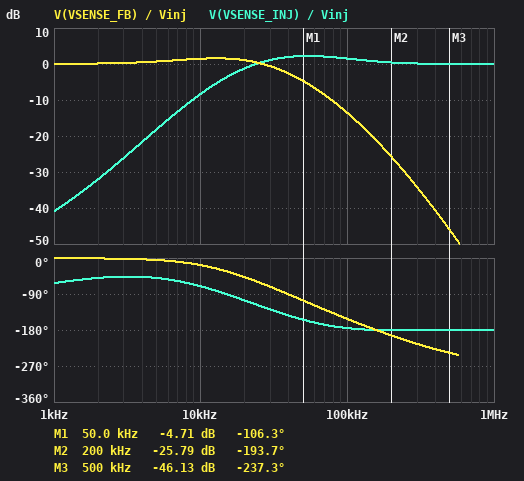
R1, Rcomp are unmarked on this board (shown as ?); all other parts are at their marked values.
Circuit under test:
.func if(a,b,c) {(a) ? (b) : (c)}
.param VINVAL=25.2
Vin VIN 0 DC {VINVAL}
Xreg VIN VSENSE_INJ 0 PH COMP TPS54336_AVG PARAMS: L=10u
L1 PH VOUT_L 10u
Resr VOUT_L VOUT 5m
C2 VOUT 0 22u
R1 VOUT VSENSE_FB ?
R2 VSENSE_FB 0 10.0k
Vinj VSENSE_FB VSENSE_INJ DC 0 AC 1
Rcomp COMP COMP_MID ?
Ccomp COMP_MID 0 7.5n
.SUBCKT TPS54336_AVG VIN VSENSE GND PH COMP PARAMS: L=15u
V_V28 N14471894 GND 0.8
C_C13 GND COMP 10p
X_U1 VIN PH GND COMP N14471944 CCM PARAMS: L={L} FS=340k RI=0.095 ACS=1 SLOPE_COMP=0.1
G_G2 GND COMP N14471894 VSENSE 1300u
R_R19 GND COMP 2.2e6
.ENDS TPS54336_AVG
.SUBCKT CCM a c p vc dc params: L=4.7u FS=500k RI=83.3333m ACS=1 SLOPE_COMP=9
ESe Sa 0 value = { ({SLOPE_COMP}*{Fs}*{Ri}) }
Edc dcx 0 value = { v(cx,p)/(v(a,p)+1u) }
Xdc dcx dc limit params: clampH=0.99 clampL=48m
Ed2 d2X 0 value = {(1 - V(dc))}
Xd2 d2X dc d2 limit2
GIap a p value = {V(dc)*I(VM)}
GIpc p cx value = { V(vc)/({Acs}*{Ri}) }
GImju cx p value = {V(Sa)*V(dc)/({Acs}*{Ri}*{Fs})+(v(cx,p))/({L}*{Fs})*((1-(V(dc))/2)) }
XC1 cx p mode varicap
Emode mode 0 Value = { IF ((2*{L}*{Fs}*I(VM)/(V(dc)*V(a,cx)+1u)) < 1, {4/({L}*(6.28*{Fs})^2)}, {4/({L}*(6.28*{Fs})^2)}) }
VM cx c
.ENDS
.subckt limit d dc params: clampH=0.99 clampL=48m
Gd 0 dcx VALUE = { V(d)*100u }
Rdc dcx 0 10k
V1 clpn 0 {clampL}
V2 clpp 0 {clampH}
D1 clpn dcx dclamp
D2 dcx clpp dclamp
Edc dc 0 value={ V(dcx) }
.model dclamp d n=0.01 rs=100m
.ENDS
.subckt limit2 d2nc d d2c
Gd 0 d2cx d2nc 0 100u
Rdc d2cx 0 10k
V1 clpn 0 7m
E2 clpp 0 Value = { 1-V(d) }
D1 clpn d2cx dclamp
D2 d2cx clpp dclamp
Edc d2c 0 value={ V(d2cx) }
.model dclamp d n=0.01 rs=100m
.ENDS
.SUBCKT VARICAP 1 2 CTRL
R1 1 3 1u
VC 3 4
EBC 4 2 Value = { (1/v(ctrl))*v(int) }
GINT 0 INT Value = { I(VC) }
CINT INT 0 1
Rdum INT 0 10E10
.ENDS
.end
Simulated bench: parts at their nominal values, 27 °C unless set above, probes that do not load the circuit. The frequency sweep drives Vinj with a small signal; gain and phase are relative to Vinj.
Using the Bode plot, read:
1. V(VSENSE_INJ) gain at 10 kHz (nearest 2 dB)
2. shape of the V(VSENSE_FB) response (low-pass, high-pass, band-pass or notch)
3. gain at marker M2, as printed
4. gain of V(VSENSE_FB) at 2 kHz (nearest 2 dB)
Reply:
-8 dB
low-pass
-25.79 dB
0 dB
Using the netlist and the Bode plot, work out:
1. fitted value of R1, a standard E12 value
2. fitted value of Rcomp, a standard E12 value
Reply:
100 kΩ
2.7 kΩ
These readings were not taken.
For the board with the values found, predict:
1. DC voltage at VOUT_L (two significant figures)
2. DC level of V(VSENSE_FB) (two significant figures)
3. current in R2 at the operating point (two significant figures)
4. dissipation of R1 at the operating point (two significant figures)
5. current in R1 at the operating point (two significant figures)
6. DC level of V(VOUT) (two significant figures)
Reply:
8.8 V
800 mV
80 µA
640 µW
80 µA
8.8 V
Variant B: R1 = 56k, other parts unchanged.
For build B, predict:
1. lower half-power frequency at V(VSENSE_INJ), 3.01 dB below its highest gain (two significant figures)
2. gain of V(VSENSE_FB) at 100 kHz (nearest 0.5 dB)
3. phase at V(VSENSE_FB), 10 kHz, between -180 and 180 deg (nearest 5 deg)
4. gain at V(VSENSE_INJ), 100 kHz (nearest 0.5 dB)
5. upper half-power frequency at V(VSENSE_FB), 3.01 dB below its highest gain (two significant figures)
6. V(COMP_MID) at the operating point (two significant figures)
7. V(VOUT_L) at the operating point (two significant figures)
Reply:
34 kHz
-9.5 dB
-10 deg
2.5 dB
59 kHz
130 mV
5.3 V
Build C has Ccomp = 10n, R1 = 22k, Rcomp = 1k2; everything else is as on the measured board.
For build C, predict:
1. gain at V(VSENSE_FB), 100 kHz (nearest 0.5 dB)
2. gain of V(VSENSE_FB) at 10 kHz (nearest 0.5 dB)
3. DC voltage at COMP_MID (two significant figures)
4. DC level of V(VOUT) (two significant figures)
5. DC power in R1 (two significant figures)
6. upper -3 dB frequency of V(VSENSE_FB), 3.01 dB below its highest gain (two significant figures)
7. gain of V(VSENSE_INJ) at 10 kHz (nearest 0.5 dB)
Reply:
-11.5 dB
1.0 dB
69 mV
2.6 V
140 µW
50 kHz
-14.5 dB
